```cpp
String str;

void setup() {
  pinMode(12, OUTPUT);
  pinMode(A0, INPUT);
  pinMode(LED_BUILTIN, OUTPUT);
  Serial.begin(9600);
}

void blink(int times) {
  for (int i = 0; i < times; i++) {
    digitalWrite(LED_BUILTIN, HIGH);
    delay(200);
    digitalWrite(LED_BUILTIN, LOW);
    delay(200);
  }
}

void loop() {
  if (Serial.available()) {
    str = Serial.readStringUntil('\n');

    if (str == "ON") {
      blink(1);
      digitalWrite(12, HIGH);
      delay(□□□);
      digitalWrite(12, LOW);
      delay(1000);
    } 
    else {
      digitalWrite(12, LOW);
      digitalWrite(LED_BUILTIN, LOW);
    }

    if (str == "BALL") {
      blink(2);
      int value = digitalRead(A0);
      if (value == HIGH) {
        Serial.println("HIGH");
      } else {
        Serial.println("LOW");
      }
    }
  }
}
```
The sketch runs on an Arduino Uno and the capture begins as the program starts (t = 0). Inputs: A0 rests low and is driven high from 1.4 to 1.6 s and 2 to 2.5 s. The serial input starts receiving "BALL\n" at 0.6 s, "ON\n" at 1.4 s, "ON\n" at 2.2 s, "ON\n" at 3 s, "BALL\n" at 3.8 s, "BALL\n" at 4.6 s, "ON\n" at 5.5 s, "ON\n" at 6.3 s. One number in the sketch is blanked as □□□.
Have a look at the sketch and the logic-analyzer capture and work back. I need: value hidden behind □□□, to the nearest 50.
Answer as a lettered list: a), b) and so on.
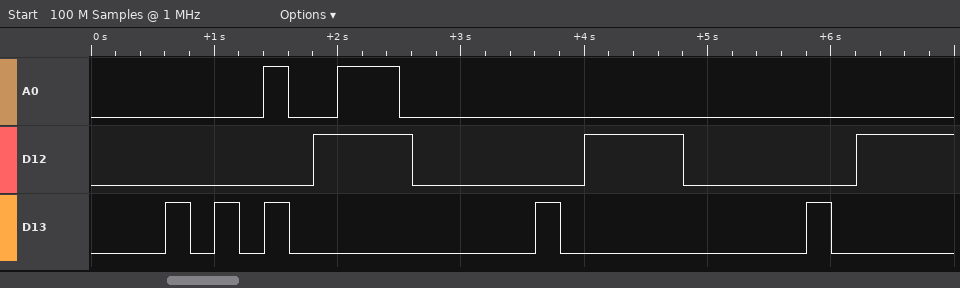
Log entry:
a) 800
